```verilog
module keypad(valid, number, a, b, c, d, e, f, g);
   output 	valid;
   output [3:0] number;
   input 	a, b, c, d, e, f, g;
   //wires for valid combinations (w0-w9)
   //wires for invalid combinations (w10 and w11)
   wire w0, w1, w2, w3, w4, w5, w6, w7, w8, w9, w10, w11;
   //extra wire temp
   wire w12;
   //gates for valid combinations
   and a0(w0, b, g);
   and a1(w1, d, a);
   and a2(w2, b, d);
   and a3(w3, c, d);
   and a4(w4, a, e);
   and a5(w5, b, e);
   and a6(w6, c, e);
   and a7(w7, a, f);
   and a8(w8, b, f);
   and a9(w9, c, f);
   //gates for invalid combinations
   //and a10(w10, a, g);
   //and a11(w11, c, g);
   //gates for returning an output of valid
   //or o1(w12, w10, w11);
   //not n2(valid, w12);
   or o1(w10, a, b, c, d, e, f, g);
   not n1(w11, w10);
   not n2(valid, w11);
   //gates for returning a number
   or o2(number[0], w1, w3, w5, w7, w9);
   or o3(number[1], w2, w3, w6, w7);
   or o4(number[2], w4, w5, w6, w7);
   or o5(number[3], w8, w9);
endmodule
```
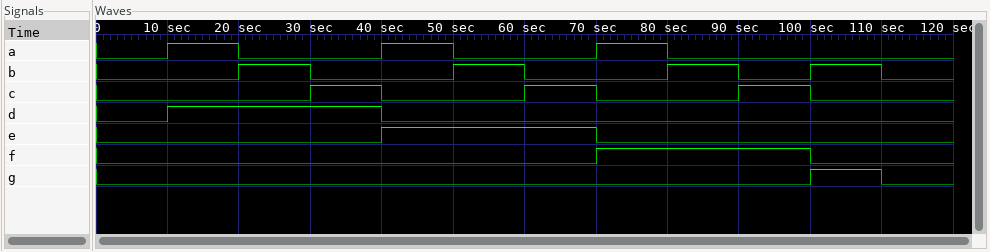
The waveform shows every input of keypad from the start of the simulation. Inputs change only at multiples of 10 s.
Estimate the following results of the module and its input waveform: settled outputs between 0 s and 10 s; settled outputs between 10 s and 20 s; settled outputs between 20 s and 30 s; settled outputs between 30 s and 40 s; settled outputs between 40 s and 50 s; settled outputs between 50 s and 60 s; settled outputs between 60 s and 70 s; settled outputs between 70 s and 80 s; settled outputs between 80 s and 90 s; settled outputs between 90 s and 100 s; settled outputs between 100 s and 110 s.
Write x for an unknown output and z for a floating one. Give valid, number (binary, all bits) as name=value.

valid=0, number=0000
valid=1, number=0001
valid=1, number=0010
valid=1, number=0011
valid=1, number=0100
valid=1, number=0101
valid=1, number=0110
valid=1, number=0111
valid=1, number=1000
valid=1, number=1001
valid=1, number=0000
